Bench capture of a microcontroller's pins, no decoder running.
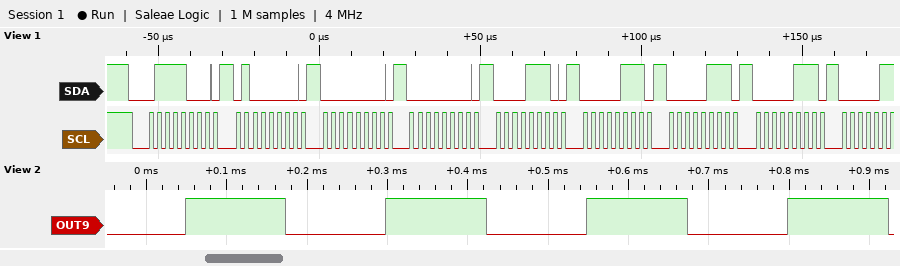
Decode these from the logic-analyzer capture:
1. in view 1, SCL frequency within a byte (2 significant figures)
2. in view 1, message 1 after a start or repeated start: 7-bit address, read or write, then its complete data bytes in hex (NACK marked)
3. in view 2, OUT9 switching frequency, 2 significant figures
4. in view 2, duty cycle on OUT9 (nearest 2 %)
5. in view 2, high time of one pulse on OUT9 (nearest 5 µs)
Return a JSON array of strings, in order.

["400 kHz", "0x3C write: 40 00 00 0E 07 07 07", "4.0 kHz", "50 %", "125 µs"]
